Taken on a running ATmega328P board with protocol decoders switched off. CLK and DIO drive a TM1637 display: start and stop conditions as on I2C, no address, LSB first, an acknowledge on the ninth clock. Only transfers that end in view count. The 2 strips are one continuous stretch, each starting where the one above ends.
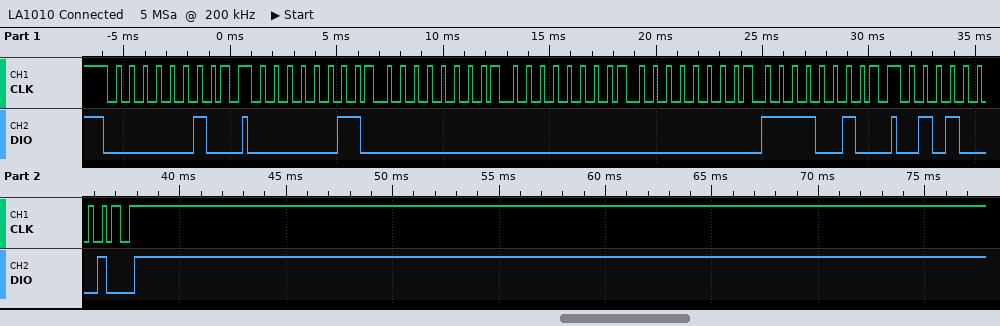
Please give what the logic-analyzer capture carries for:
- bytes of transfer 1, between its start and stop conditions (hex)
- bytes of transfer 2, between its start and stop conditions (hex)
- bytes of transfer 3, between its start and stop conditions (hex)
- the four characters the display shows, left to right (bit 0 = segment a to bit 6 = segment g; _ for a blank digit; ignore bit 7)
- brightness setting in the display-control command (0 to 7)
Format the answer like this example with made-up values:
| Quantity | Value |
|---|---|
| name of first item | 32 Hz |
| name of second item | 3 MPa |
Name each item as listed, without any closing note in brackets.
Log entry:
| Quantity | Value |
|---|---|
| bytes of transfer 1, between its start and stop conditions | 40 |
| bytes of transfer 2, between its start and stop conditions | C0 00 00 00 4F |
| bytes of transfer 3, between its start and stop conditions | 8A |
| the four characters the display shows, left to right | ___3 |
| brightness setting in the display-control command | 2 |
